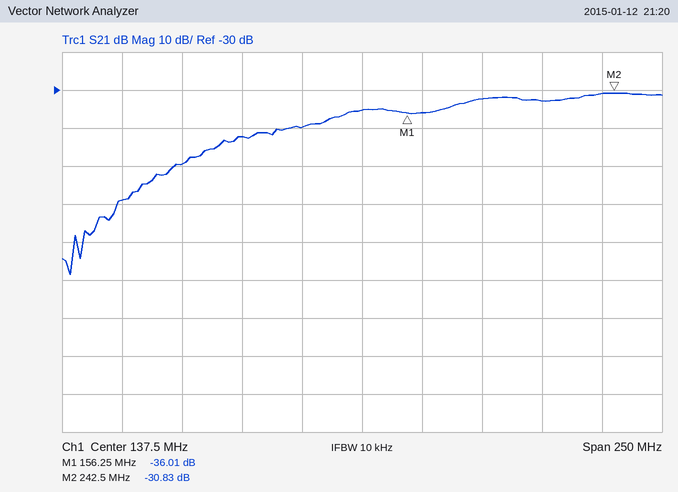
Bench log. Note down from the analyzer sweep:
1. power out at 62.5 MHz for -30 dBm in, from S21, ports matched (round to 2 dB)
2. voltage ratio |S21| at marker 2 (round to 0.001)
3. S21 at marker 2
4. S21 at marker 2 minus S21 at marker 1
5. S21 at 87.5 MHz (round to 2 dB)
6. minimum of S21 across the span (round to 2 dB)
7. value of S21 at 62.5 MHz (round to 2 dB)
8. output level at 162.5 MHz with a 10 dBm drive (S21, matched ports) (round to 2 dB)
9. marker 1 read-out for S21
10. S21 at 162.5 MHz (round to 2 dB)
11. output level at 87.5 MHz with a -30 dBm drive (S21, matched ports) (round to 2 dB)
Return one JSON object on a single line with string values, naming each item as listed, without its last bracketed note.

{"power out at 62.5 MHz for -30 dBm in, from S21, ports matched": "-80 dBm", "voltage ratio |S21| at marker 2": "0.029", "S21 at marker 2": "-30.83 dB", "S21 at marker 2 minus S21 at marker 1": "5.18 dB", "S21 at 87.5 MHz": "-42 dB", "minimum of S21 across the span": "-78 dB", "value of S21 at 62.5 MHz": "-50 dB", "output level at 162.5 MHz with a 10 dBm drive (S21, matched ports)": "-26 dBm", "marker 1 read-out for S21": "-36.01 dB", "S21 at 162.5 MHz": "-36 dB", "output level at 87.5 MHz with a -30 dBm drive (S21, matched ports)": "-72 dBm"}
